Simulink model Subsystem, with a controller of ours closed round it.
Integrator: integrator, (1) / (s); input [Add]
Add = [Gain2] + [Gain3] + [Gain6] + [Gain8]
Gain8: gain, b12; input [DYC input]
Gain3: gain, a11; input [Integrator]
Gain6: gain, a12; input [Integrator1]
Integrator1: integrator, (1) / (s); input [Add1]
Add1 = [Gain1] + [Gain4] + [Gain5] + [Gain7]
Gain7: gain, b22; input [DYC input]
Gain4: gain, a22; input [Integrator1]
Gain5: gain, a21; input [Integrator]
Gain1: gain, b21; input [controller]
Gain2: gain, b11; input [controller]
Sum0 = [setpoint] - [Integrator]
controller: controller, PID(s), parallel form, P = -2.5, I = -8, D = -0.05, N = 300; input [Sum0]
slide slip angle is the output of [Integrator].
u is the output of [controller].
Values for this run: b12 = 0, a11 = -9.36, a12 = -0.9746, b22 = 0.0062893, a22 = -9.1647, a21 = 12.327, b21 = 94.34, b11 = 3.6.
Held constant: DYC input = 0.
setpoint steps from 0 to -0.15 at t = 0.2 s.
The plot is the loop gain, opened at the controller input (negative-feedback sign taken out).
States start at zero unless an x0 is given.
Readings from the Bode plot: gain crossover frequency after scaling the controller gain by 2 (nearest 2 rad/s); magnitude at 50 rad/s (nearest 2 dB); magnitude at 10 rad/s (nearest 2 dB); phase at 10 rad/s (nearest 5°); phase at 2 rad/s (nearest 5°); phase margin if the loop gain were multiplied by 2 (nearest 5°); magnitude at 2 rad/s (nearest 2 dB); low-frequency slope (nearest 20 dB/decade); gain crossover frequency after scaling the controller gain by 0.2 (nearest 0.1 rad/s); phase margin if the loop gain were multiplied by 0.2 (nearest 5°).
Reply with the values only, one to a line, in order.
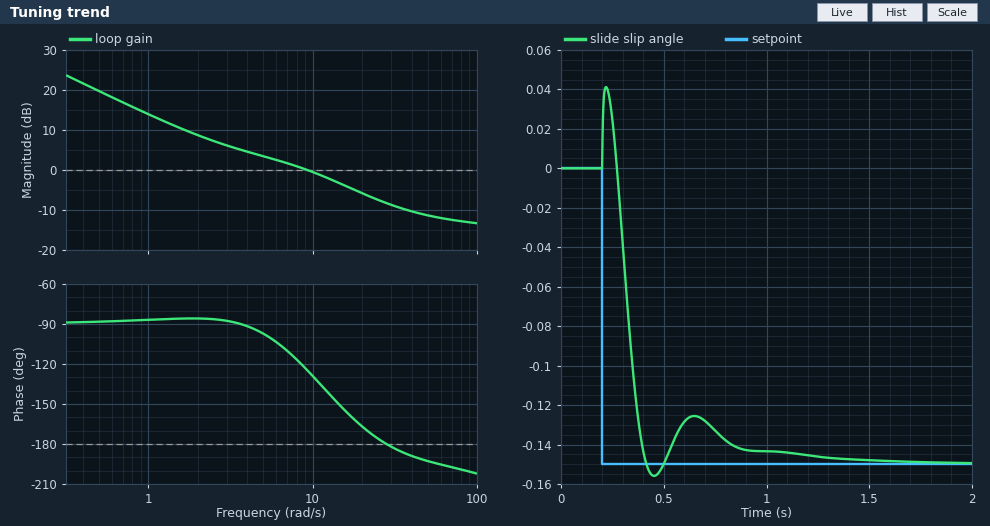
20 rad/s
-12 dB
0 dB
-130°
-85°
10°
8 dB
-20 dB/decade
1.0 rad/s
95°
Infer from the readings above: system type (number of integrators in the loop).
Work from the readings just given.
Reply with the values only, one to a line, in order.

1
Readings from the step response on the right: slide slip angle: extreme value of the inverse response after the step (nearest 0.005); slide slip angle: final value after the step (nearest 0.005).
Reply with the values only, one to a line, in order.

0.040
-0.150
